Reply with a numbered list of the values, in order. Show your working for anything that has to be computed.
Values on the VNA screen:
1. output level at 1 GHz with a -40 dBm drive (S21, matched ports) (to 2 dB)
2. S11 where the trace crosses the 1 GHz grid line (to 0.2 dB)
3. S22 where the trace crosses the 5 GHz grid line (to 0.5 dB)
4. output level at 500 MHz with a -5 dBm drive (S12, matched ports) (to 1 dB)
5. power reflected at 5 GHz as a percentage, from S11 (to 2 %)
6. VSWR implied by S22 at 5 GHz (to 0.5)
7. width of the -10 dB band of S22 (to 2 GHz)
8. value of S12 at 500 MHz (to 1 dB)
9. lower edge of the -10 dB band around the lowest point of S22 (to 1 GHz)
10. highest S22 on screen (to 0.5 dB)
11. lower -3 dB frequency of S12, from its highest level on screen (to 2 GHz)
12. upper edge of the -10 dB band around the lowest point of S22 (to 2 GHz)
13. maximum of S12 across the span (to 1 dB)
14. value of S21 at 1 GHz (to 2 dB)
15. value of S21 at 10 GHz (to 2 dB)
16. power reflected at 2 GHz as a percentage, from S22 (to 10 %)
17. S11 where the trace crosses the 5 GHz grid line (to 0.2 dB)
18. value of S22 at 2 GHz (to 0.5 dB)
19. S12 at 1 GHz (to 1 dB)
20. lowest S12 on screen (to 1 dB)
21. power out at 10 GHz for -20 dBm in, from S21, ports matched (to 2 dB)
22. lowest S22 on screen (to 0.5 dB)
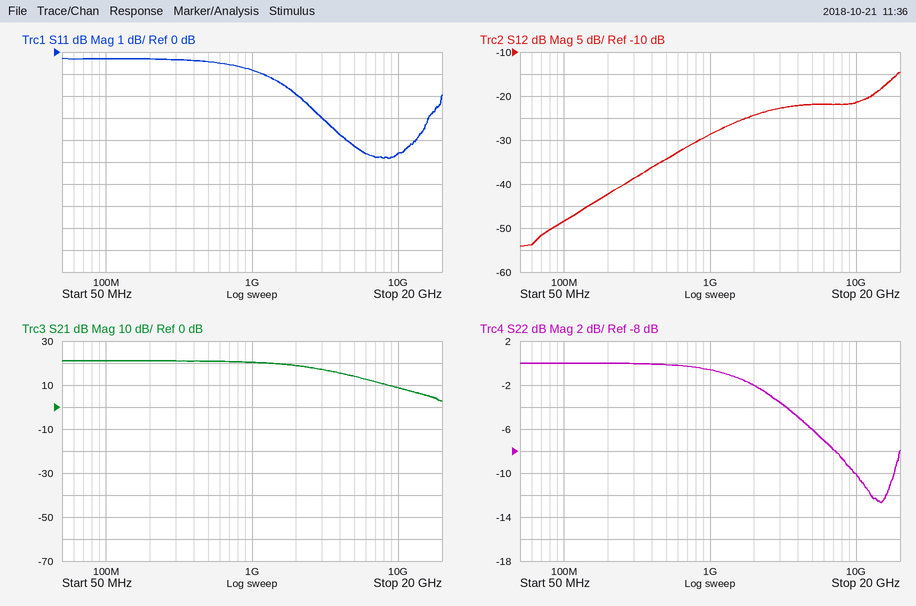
1. -40 dBm + (20 dB) = -20 dBm
2. -0.8 dB
3. -6.0 dB
4. -5 dBm + (-34 dB) = -39 dBm
5. 10^(-4.2/10) ≈ 38 %
6. |Γ| = 10^(-6/20) = 0.5012; VSWR = (1 + 0.5012)/(1 − 0.5012) ≈ 3.0
7. 18 GHz − 10 GHz = 8 GHz
8. -34 dB
9. 10 GHz
10. 0.0 dB
11. 16 GHz
12. 18 GHz
13. -15 dB
14. 20 dB
15. 8 dB
16. 10^(-2/10) ≈ 63.1 %, so 60 % to the nearest 10 %
17. -4.2 dB
18. -2.0 dB
19. -29 dB
20. -54 dB
21. -20 dBm + (8 dB) = -12 dBm
22. -12.5 dB
